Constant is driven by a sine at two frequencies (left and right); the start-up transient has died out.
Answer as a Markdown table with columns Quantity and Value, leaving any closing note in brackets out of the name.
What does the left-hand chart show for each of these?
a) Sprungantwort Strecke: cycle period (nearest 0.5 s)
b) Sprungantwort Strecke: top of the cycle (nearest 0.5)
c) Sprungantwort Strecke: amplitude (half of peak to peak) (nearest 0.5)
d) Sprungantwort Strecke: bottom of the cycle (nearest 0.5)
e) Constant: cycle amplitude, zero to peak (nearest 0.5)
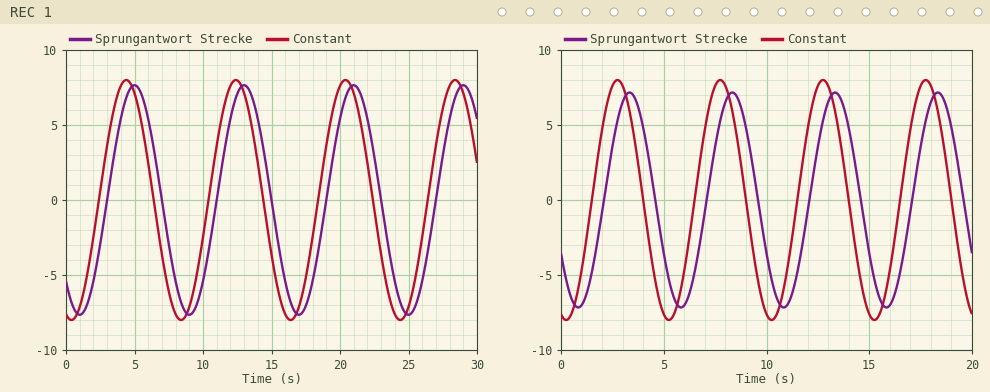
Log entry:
| Quantity | Value |
|---|---|
| Sprungantwort Strecke: cycle period | 8.0 s |
| Sprungantwort Strecke: top of the cycle | 7.5 |
| Sprungantwort Strecke: amplitude (half of peak to peak) | 7.5 |
| Sprungantwort Strecke: bottom of the cycle | -7.5 |
| Constant: cycle amplitude, zero to peak | 8.0 |
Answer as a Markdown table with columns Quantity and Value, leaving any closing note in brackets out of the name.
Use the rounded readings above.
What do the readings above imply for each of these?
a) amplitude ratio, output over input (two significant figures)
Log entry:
| Quantity | Value |
|---|---|
| amplitude ratio, output over input | 0.94 |
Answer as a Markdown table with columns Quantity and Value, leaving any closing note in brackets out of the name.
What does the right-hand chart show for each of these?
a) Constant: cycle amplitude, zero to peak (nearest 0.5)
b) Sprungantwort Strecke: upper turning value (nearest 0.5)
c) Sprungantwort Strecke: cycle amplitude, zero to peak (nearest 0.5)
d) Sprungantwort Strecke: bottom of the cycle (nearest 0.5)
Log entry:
| Quantity | Value |
|---|---|
| Constant: cycle amplitude, zero to peak | 8.0 |
| Sprungantwort Strecke: upper turning value | 7.0 |
| Sprungantwort Strecke: cycle amplitude, zero to peak | 7.0 |
| Sprungantwort Strecke: bottom of the cycle | -7.0 |
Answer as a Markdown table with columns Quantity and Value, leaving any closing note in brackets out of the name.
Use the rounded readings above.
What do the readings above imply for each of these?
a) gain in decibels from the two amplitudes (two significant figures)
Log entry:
| Quantity | Value |
|---|---|
| gain in decibels from the two amplitudes | -1.2 dB |
